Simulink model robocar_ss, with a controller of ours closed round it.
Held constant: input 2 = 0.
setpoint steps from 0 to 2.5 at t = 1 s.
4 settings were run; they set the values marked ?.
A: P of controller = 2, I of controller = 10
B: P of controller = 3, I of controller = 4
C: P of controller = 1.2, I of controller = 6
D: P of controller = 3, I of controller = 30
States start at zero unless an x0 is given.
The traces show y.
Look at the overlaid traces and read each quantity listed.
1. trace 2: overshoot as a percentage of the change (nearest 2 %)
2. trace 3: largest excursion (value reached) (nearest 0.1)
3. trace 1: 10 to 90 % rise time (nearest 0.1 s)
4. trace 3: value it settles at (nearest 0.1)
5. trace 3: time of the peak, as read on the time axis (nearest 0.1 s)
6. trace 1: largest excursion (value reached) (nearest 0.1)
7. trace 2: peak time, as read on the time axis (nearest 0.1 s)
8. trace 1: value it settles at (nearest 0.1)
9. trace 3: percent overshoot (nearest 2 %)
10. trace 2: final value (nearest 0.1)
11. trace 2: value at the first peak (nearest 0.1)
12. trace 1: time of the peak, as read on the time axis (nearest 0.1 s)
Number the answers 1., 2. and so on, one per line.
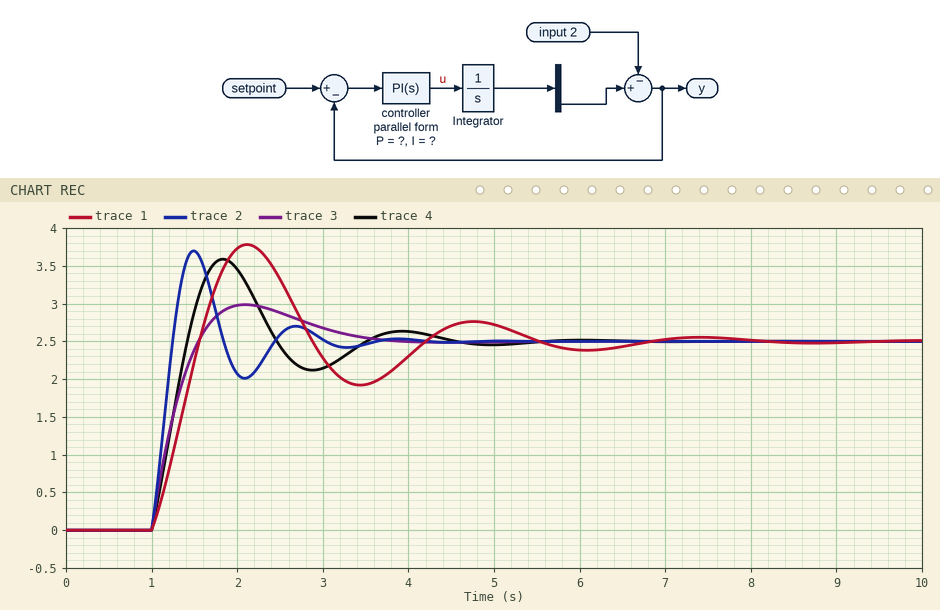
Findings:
1. 48 %
2. 3.0
3. 0.4 s
4. 2.5
5. 2.1 s
6. 3.8
7. 1.5 s
8. 2.5
9. 20 %
10. 2.5
11. 3.7
12. 2.1 s
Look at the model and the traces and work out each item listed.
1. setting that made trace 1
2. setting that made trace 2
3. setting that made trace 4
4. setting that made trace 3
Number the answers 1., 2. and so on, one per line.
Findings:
1. C
2. D
3. A
4. B
